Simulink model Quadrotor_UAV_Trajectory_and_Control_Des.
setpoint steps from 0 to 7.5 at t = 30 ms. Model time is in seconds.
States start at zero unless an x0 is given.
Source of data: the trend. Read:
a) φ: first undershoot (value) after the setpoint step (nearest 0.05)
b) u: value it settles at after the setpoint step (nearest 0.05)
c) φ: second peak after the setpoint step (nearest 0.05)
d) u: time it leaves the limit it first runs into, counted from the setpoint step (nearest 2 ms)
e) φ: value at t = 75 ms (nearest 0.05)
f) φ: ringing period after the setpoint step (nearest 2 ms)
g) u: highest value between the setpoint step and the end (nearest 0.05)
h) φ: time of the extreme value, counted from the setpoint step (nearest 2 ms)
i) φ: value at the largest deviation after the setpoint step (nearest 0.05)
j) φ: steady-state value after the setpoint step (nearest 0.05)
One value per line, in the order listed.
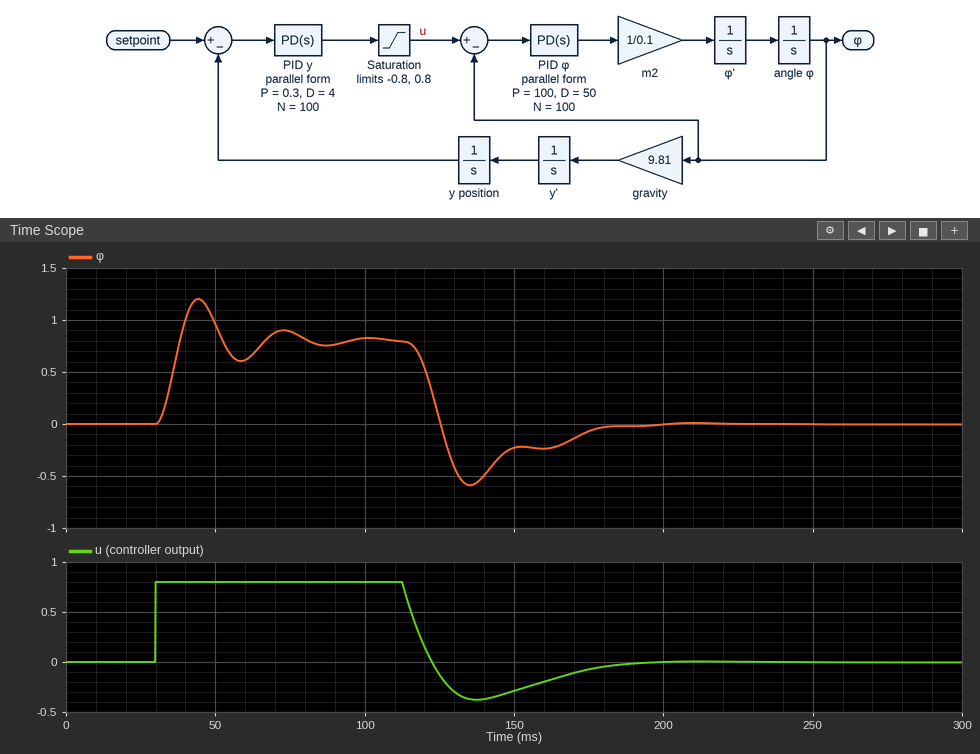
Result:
0.60
0.00
0.90
82 ms
0.90
28 ms
0.80
14 ms
1.20
0.00
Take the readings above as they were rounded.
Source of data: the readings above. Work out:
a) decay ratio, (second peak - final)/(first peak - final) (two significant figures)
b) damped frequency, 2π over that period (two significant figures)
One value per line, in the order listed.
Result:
0.75
0.22 rad/ms
